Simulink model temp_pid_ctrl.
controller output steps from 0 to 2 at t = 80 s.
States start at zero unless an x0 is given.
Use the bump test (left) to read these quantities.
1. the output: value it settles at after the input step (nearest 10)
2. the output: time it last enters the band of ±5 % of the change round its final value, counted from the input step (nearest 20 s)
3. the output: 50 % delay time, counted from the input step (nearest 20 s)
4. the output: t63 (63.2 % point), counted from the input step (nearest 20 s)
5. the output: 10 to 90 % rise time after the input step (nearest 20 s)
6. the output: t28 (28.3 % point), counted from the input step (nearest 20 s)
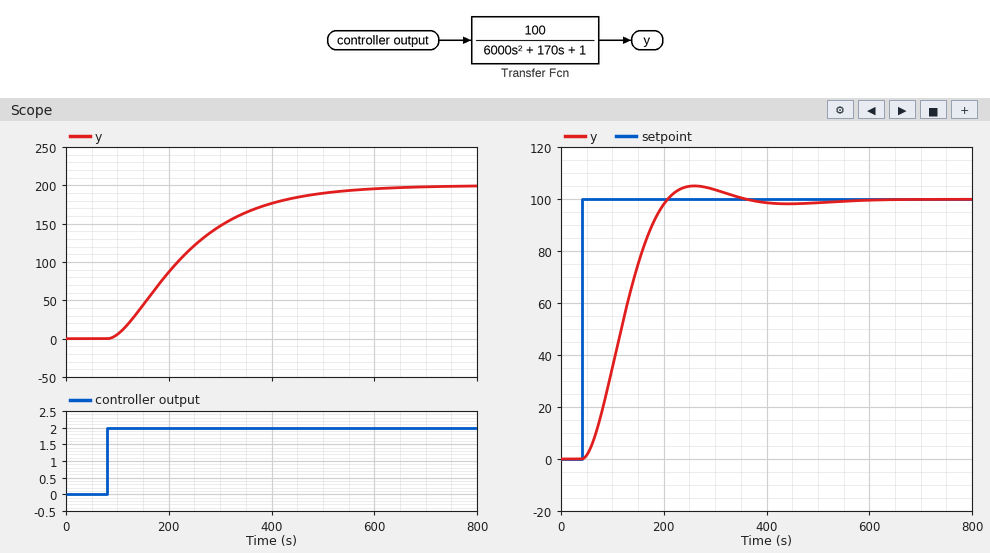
200
420 s
140 s
180 s
300 s
80 s
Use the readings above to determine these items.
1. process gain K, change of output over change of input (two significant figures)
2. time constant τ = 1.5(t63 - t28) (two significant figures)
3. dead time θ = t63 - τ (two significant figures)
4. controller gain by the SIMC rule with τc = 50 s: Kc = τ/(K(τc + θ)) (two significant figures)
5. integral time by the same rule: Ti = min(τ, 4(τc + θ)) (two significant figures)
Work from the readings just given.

100
150 s
30 s
0.019
150 s
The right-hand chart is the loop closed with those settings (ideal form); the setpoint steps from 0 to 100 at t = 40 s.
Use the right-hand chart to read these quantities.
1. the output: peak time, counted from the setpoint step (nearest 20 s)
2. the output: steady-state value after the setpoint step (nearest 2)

220 s
100
